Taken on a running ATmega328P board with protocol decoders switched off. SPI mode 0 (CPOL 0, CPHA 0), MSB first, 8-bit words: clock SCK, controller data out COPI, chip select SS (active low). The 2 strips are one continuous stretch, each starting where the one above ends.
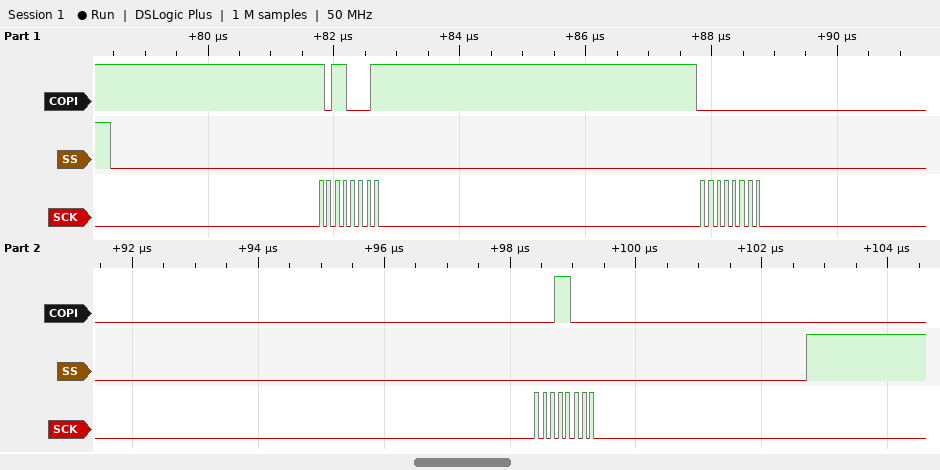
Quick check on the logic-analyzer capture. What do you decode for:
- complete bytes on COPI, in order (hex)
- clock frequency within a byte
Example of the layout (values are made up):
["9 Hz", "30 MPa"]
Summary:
["0xB1 0x00 0x18", "8 MHz"]
